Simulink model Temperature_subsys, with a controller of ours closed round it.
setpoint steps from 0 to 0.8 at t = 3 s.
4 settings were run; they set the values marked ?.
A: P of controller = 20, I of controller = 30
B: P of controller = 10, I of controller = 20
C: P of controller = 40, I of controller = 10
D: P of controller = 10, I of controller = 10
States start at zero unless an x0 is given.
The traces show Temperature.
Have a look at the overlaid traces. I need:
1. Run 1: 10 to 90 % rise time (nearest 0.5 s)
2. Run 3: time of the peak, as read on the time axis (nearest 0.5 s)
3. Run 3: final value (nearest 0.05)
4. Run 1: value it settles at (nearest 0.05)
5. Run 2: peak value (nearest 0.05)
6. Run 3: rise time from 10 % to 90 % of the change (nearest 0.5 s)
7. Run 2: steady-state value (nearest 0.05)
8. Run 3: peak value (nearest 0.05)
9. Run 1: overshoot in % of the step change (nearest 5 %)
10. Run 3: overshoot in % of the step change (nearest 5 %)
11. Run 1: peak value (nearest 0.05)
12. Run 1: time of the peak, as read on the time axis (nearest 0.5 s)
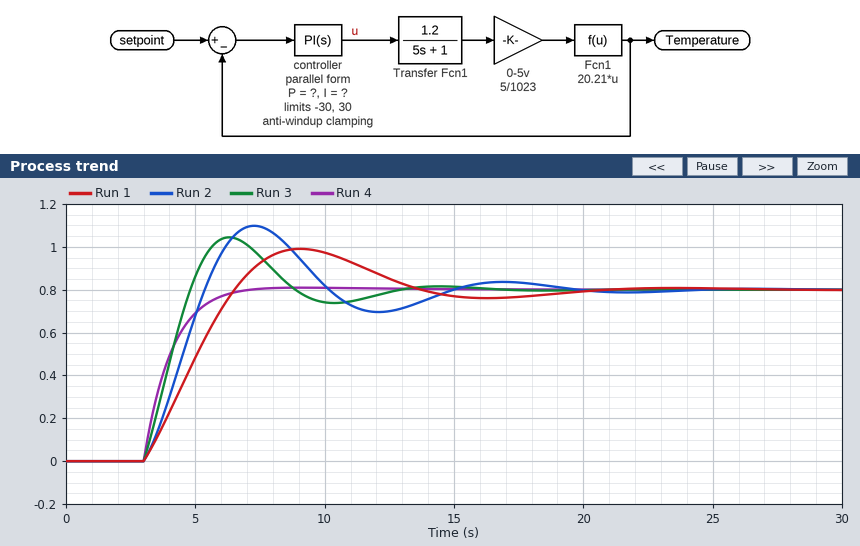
2.5 s
6.5 s
0.80
0.80
1.10
1.5 s
0.80
1.05
25 %
30 %
1.00
9.0 s
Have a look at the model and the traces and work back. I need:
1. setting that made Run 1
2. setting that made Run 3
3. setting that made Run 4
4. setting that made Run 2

D
A
C
B
